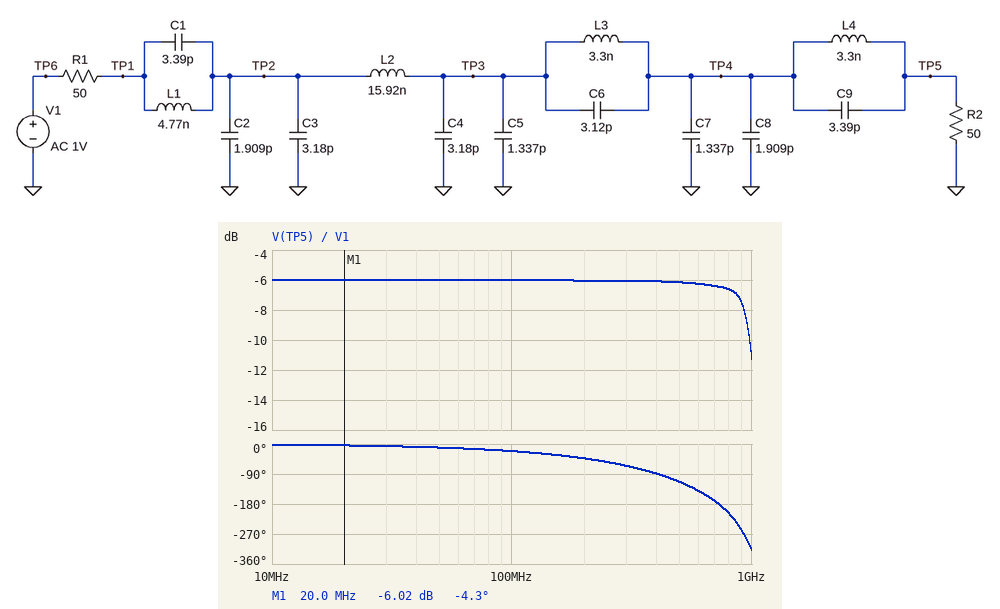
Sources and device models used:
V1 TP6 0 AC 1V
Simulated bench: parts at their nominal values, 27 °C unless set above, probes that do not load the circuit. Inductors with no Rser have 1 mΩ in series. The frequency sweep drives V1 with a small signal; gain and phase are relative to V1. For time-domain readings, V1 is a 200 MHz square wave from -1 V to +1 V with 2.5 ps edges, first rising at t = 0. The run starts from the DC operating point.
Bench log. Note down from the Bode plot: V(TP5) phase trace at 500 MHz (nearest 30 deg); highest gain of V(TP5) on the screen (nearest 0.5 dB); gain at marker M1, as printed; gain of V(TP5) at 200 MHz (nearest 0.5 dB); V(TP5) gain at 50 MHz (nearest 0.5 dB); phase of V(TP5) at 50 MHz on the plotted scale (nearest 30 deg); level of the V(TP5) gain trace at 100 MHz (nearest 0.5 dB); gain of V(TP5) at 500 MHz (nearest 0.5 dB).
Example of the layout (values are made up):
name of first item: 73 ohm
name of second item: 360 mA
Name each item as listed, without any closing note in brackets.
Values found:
V(TP5) phase trace at 500 MHz: -120 deg
highest gain of V(TP5) on the screen: -6.0 dB
gain at marker M1, as printed: -6.02 dB
gain of V(TP5) at 200 MHz: -6.0 dB
V(TP5) gain at 50 MHz: -6.0 dB
phase of V(TP5) at 50 MHz on the plotted scale: 0 deg
level of the V(TP5) gain trace at 100 MHz: -6.0 dB
gain of V(TP5) at 500 MHz: -6.0 dB
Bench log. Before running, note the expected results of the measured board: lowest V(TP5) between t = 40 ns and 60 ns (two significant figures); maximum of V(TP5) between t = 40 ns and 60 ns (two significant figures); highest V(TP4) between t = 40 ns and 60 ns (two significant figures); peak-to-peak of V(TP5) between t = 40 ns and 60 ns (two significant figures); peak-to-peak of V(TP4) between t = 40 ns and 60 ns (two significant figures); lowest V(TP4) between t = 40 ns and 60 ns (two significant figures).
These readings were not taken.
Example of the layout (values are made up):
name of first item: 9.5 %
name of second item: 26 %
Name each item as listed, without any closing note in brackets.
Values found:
lowest V(TP5) between t = 40 ns and 60 ns: -680 mV
maximum of V(TP5) between t = 40 ns and 60 ns: 680 mV
highest V(TP4) between t = 40 ns and 60 ns: 690 mV
peak-to-peak of V(TP5) between t = 40 ns and 60 ns: 1.4 V
peak-to-peak of V(TP4) between t = 40 ns and 60 ns: 1.4 V
lowest V(TP4) between t = 40 ns and 60 ns: -690 mV
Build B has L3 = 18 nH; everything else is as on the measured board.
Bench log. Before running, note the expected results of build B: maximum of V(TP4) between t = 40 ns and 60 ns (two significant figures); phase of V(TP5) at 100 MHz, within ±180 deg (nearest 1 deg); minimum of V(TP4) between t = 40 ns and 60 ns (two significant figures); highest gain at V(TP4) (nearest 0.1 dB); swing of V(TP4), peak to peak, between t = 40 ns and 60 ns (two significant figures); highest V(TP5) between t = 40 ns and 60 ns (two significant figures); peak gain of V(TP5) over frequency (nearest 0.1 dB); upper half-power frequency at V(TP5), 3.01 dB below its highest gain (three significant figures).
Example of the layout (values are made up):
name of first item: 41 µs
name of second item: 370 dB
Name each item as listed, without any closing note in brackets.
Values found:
maximum of V(TP4) between t = 40 ns and 60 ns: 640 mV
phase of V(TP5) at 100 MHz, within ±180 deg: -27 deg
minimum of V(TP4) between t = 40 ns and 60 ns: -640 mV
highest gain at V(TP4): -6.0 dB
swing of V(TP4), peak to peak, between t = 40 ns and 60 ns: 1.3 V
highest V(TP5) between t = 40 ns and 60 ns: 630 mV
peak gain of V(TP5) over frequency: -6.0 dB
upper half-power frequency at V(TP5), 3.01 dB below its highest gain: 506 MHz
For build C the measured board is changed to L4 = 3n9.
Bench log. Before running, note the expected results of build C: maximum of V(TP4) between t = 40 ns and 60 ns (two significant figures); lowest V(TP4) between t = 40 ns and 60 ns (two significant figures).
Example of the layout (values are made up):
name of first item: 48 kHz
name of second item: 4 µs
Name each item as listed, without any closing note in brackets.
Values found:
maximum of V(TP4) between t = 40 ns and 60 ns: 710 mV
lowest V(TP4) between t = 40 ns and 60 ns: -710 mV
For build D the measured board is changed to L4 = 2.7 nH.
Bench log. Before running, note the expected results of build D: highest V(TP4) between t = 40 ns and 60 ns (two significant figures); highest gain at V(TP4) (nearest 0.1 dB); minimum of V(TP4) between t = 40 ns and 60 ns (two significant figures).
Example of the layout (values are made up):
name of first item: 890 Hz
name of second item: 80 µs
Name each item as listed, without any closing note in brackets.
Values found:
highest V(TP4) between t = 40 ns and 60 ns: 680 mV
highest gain at V(TP4): -6.0 dB
minimum of V(TP4) between t = 40 ns and 60 ns: -680 mV
